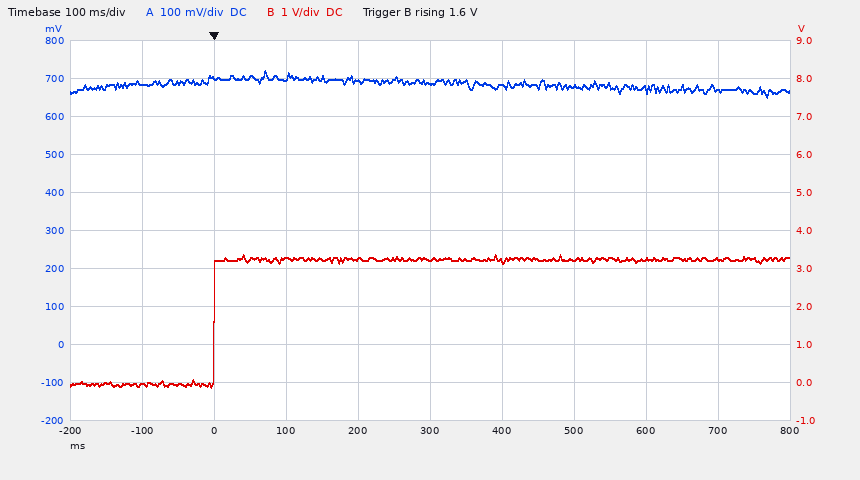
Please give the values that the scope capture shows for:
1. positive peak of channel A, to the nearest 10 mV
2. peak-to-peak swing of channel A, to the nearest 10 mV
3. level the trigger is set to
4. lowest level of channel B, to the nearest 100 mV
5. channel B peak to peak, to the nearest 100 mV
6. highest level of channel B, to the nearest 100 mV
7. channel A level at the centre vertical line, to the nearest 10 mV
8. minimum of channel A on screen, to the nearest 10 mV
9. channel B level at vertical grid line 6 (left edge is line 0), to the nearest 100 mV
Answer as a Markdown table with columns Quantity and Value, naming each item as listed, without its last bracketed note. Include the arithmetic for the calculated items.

| Quantity | Value |
|---|---|
| positive peak of channel A, to the nearest 10 mV | 720 mV |
| peak-to-peak swing of channel A, to the nearest 10 mV | 720 mV − (650 mV) = 70 mV |
| level the trigger is set to | 1.6 V |
| lowest level of channel B, to the nearest 100 mV | -100 mV |
| channel B peak to peak, to the nearest 100 mV | 3.4 V − (-100 mV) = 3.5 V |
| highest level of channel B, to the nearest 100 mV | 3.4 V |
| channel A level at the centre vertical line, to the nearest 10 mV | 690 mV |
| minimum of channel A on screen, to the nearest 10 mV | 650 mV |
| channel B level at vertical grid line 6 (left edge is line 0), to the nearest 100 mV | 3.2 V |
